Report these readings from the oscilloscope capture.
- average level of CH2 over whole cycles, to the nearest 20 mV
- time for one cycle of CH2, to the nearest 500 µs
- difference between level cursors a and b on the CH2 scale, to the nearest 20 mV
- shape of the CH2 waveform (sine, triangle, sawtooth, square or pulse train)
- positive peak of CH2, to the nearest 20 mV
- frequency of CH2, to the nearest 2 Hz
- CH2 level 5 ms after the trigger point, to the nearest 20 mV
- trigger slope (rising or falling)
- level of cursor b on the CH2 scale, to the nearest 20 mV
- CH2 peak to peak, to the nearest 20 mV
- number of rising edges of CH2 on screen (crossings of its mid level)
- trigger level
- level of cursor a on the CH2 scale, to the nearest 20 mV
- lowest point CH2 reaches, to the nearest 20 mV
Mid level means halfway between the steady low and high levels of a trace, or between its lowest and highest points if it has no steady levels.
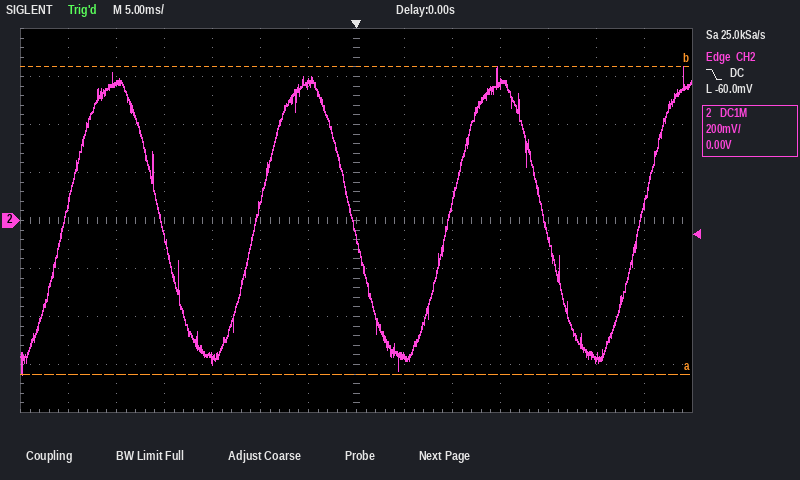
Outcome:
0 mV
20.0 ms
1.28 V
sine
640 mV
50 Hz
-560 mV
falling
640 mV
1.28 V
4
-60.0 mV
-640 mV
-640 mV
